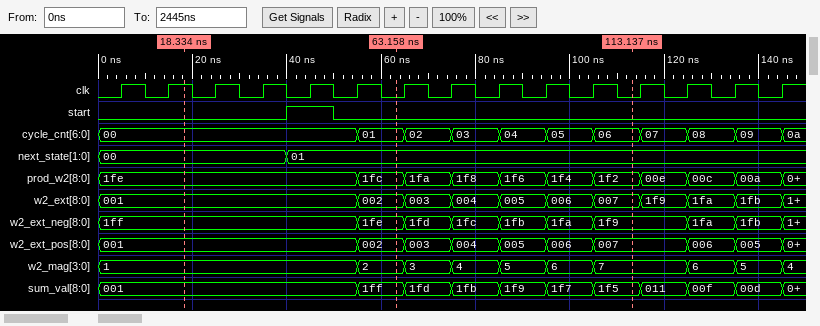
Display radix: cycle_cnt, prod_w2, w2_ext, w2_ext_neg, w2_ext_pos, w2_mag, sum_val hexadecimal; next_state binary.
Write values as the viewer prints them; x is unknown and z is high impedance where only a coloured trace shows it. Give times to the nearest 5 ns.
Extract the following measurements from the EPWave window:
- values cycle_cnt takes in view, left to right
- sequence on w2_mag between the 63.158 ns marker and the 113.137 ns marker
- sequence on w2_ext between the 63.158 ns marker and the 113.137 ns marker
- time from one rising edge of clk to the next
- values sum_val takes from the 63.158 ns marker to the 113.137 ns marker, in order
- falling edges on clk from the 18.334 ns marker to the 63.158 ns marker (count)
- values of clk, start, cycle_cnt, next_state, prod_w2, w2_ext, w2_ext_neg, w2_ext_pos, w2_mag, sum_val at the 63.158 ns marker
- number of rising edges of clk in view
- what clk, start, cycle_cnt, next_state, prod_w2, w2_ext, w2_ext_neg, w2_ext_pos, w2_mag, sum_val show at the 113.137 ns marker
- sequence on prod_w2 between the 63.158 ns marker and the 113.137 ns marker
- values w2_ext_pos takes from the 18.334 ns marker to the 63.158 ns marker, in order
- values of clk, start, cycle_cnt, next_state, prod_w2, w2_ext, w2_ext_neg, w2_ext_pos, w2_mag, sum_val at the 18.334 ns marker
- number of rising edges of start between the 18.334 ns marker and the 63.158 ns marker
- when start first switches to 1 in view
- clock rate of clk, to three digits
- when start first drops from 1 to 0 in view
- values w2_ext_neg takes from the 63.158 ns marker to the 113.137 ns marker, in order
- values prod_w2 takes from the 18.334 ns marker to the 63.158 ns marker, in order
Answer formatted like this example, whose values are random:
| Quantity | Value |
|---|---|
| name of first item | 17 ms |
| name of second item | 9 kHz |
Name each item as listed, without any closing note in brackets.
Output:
| Quantity | Value |
|---|---|
| values cycle_cnt takes in view, left to right | 00, 01, 02, 03, 04, 05, 06, 07, 08, 09, 0a |
| sequence on w2_mag between the 63.158 ns marker and the 113.137 ns marker | 2, 3, 4, 5, 6, 7 |
| sequence on w2_ext between the 63.158 ns marker and the 113.137 ns marker | 002, 003, 004, 005, 006, 007 |
| time from one rising edge of clk to the next | 10 ns |
| values sum_val takes from the 63.158 ns marker to the 113.137 ns marker, in order | 1ff, 1fd, 1fb, 1f9, 1f7, 1f5 |
| falling edges on clk from the 18.334 ns marker to the 63.158 ns marker | 5 |
| values of clk, start, cycle_cnt, next_state, prod_w2, w2_ext, w2_ext_neg, w2_ext_pos, w2_mag, sum_val at the 63.158 ns marker | clk=0, start=0, cycle_cnt=01, next_state=01, prod_w2=1fc, w2_ext=002, w2_ext_neg=1fe, w2_ext_pos=002, w2_mag=2, sum_val=1ff |
| number of rising edges of clk in view | 15 |
| what clk, start, cycle_cnt, next_state, prod_w2, w2_ext, w2_ext_neg, w2_ext_pos, w2_mag, sum_val show at the 113.137 ns marker | clk=0, start=0, cycle_cnt=06, next_state=01, prod_w2=1f2, w2_ext=007, w2_ext_neg=1f9, w2_ext_pos=007, w2_mag=7, sum_val=1f5 |
| sequence on prod_w2 between the 63.158 ns marker and the 113.137 ns marker | 1fc, 1fa, 1f8, 1f6, 1f4, 1f2 |
| values w2_ext_pos takes from the 18.334 ns marker to the 63.158 ns marker, in order | 001, 002 |
| values of clk, start, cycle_cnt, next_state, prod_w2, w2_ext, w2_ext_neg, w2_ext_pos, w2_mag, sum_val at the 18.334 ns marker | clk=1, start=0, cycle_cnt=00, next_state=00, prod_w2=1fe, w2_ext=001, w2_ext_neg=1ff, w2_ext_pos=001, w2_mag=1, sum_val=001 |
| number of rising edges of start between the 18.334 ns marker and the 63.158 ns marker | 1 |
| when start first switches to 1 in view | 40 ns |
| clock rate of clk, to three digits | 100 MHz |
| when start first drops from 1 to 0 in view | 50 ns |
| values w2_ext_neg takes from the 63.158 ns marker to the 113.137 ns marker, in order | 1fe, 1fd, 1fc, 1fb, 1fa, 1f9 |
| values prod_w2 takes from the 18.334 ns marker to the 63.158 ns marker, in order | 1fe, 1fc |
